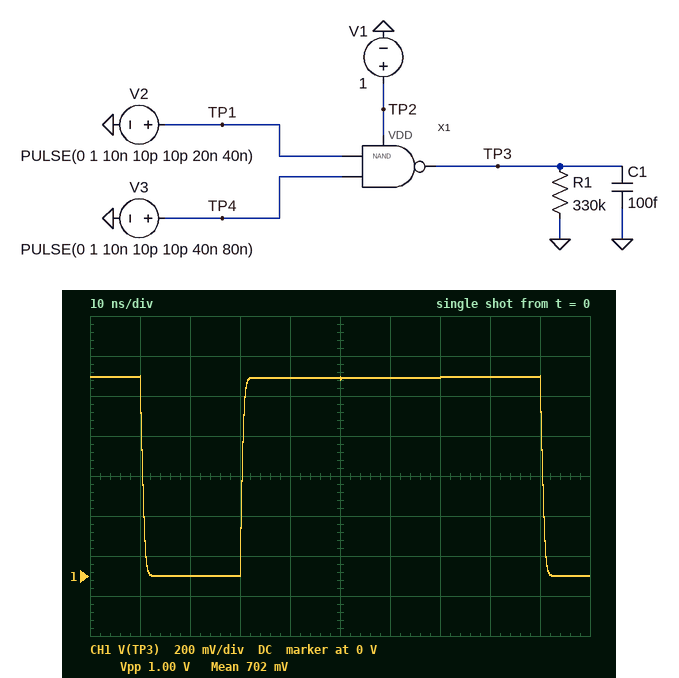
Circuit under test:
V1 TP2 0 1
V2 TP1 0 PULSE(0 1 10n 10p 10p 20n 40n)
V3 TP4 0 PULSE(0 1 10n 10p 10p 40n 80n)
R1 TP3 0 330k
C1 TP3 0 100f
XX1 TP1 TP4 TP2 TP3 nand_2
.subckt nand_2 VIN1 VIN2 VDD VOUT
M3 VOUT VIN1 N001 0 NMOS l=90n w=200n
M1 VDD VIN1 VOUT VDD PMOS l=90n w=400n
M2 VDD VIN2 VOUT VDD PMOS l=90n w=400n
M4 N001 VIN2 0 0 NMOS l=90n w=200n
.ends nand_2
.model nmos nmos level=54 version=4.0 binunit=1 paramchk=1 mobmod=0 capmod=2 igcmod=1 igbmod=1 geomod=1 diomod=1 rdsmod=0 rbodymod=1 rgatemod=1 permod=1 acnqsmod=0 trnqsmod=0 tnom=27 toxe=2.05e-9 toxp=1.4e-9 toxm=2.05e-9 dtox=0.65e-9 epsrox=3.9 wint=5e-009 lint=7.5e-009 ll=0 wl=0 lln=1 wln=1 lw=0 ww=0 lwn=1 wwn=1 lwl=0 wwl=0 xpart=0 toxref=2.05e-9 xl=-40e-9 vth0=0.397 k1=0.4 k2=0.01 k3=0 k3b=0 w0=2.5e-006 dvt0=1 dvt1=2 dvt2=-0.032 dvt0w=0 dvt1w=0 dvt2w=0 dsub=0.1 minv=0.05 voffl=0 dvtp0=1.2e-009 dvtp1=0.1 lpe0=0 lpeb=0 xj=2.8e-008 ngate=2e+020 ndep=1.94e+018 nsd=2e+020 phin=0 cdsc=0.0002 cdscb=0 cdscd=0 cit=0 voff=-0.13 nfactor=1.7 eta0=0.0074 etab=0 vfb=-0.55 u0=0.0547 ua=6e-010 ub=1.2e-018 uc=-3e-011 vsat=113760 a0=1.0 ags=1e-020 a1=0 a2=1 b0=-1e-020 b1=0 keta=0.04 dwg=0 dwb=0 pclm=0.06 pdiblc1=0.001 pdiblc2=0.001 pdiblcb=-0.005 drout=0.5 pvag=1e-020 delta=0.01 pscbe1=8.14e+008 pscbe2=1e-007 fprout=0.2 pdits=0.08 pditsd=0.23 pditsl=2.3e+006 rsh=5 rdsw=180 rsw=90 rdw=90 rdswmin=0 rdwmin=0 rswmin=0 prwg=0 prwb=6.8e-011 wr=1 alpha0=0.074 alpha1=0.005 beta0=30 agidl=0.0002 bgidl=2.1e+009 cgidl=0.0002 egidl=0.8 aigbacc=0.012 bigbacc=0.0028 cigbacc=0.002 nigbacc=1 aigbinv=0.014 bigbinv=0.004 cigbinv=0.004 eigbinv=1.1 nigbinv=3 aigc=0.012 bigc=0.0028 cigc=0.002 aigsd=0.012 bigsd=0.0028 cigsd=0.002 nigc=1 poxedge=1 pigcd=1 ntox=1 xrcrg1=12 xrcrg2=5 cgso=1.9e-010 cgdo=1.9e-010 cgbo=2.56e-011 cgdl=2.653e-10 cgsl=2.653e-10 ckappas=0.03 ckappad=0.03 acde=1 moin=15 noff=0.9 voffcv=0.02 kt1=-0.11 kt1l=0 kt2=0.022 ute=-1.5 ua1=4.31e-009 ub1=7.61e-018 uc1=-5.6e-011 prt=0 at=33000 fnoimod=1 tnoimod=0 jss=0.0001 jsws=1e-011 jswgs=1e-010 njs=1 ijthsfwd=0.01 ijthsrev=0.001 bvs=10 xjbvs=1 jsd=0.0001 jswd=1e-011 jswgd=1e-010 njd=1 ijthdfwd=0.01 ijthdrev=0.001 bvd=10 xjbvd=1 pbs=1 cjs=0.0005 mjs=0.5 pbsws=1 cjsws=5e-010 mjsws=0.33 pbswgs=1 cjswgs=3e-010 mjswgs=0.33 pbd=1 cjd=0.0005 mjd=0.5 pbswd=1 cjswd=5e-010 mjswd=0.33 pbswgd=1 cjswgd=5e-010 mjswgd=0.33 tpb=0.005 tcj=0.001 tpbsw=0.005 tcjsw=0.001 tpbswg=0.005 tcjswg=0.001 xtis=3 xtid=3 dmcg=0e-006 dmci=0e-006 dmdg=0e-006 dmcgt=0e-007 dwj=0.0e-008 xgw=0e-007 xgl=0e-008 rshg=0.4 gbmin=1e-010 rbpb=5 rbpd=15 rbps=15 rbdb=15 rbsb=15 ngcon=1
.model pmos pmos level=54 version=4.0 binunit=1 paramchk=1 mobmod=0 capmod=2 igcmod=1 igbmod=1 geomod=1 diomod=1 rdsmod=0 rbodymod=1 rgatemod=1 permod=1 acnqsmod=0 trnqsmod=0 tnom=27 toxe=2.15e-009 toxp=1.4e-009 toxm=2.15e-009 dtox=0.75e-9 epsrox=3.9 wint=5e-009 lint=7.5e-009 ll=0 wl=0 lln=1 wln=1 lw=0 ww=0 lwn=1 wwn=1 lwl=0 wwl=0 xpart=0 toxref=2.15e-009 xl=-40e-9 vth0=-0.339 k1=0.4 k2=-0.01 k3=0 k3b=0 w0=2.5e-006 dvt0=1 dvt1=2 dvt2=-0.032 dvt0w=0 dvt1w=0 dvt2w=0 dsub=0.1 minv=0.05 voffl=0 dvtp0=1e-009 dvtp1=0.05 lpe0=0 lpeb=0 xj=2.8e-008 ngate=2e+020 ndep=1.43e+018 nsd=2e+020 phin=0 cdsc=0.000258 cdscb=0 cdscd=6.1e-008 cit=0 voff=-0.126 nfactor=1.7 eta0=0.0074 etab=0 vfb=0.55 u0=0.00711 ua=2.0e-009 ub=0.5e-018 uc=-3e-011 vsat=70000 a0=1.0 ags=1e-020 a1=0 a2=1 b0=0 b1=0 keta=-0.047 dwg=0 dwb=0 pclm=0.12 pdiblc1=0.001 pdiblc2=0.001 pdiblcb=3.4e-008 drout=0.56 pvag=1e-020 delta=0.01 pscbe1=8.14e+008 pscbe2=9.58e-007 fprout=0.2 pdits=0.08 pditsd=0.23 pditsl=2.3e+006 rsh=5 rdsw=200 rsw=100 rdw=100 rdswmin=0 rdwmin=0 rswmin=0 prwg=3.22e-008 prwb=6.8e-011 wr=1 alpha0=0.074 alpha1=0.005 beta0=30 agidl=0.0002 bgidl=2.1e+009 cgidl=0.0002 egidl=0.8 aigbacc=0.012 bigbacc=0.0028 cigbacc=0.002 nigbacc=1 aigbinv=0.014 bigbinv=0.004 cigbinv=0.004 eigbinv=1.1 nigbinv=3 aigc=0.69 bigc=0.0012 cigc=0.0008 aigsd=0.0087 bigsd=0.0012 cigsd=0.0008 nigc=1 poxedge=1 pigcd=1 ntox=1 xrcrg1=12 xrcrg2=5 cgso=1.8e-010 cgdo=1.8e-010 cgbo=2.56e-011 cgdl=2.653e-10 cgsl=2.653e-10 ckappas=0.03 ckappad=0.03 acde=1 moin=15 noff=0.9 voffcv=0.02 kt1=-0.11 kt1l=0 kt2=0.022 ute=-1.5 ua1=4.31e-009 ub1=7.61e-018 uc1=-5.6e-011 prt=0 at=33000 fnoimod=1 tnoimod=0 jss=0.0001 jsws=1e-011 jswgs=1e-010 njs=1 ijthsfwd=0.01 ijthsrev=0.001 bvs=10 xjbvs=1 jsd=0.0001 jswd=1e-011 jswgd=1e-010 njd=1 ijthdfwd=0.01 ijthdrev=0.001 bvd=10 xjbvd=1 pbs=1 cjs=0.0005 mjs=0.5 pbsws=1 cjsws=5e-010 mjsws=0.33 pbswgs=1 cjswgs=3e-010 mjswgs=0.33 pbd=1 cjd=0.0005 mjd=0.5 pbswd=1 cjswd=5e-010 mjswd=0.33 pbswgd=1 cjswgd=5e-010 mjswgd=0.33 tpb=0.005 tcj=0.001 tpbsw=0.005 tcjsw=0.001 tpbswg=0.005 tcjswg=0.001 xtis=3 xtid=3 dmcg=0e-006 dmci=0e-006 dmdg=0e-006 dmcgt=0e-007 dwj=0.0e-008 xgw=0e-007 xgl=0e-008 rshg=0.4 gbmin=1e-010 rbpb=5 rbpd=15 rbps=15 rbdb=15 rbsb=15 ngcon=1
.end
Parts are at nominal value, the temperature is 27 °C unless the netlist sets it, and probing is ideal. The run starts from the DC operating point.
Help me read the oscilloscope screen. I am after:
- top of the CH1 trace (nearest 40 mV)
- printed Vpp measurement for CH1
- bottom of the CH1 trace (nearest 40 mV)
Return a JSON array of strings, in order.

["1.00 V", "1.00 V", "0 V"]
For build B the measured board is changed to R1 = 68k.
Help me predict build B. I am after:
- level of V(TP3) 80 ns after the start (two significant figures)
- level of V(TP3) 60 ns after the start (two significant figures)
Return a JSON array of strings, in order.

["980 mV", "960 mV"]
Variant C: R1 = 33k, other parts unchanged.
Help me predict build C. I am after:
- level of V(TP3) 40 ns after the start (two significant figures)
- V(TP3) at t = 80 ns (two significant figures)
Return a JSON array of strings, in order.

["920 mV", "960 mV"]
